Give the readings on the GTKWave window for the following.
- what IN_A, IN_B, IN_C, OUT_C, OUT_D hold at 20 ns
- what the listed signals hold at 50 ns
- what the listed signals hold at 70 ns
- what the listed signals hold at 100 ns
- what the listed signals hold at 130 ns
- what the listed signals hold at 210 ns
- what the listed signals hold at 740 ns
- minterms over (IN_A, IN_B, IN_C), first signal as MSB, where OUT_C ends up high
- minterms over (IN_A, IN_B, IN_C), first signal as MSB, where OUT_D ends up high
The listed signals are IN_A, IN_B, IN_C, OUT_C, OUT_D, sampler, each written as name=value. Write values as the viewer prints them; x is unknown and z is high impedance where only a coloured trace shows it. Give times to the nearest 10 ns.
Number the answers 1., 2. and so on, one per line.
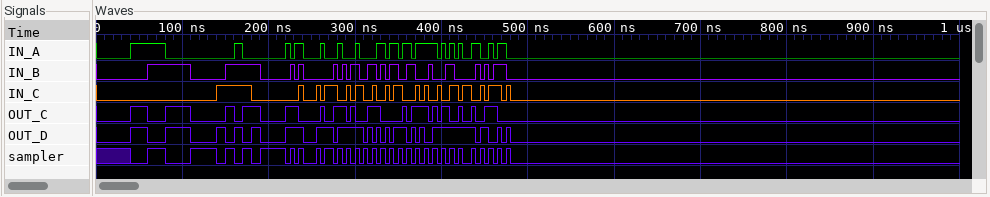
1. IN_A=0, IN_B=0, IN_C=0, OUT_C=0, OUT_D=0
2. IN_A=1, IN_B=0, IN_C=0, OUT_C=1, OUT_D=1, sampler=0
3. IN_A=1, IN_B=1, IN_C=0, OUT_C=0, OUT_D=0, sampler=1
4. IN_A=0, IN_B=1, IN_C=0, OUT_C=1, OUT_D=1, sampler=0
5. IN_A=0, IN_B=0, IN_C=0, OUT_C=0, OUT_D=0, sampler=1
6. IN_A=0, IN_B=0, IN_C=0, OUT_C=0, OUT_D=0, sampler=1
7. IN_A=0, IN_B=0, IN_C=0, OUT_C=0, OUT_D=0, sampler=0
8. 2, 3, 4, 5
9. 1, 2, 4, 7
